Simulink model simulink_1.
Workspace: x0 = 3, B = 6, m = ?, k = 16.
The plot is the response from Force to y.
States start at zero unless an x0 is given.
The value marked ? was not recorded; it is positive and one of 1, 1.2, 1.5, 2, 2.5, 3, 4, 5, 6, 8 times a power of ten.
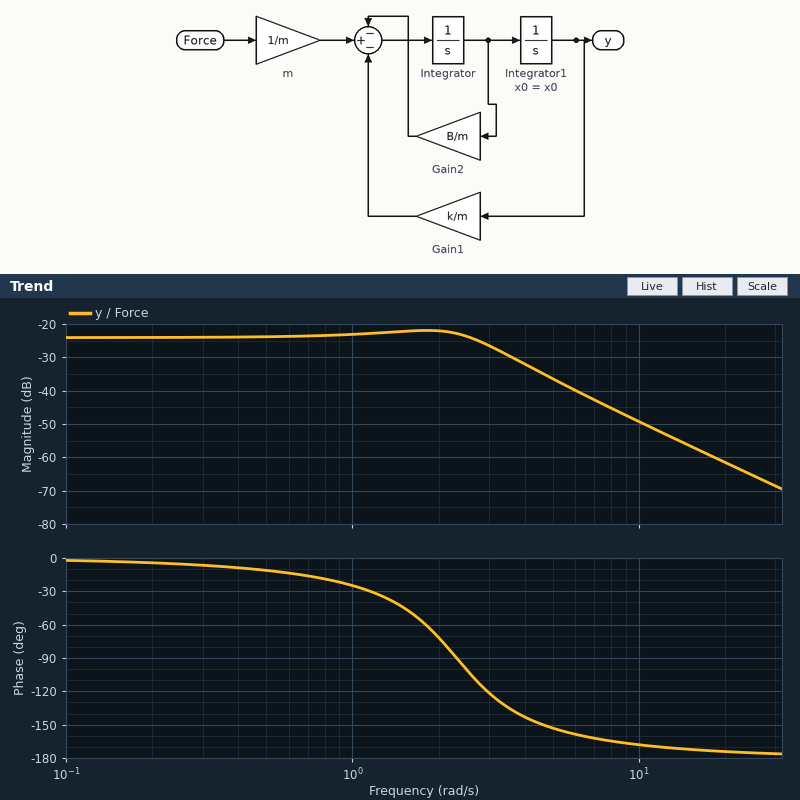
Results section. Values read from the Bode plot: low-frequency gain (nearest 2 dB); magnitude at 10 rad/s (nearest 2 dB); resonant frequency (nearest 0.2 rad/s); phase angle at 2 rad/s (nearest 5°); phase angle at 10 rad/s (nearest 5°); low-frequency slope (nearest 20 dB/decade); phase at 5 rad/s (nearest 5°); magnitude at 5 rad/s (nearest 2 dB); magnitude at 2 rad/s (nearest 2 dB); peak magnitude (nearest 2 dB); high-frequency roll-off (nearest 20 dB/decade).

-24 dB
-50 dB
1.8 rad/s
-70°
-170°
0 dB/decade
-155°
-36 dB
-22 dB
-22 dB
-40 dB/decade
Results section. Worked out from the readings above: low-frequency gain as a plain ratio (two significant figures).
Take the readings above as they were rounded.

0.063
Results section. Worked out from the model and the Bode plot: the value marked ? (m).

3
